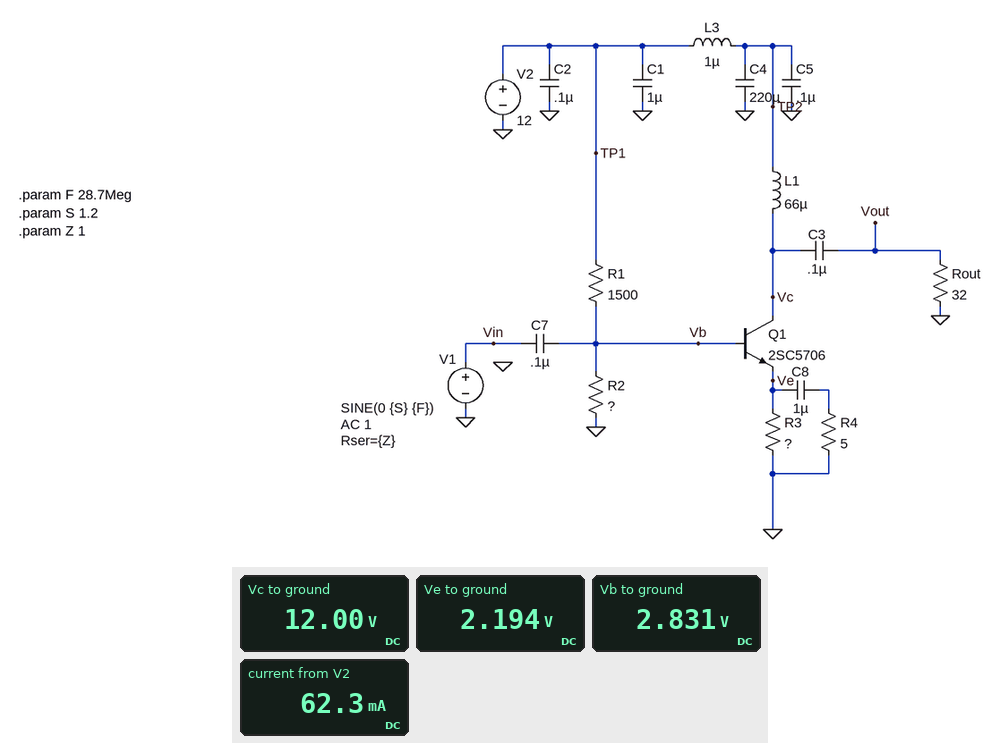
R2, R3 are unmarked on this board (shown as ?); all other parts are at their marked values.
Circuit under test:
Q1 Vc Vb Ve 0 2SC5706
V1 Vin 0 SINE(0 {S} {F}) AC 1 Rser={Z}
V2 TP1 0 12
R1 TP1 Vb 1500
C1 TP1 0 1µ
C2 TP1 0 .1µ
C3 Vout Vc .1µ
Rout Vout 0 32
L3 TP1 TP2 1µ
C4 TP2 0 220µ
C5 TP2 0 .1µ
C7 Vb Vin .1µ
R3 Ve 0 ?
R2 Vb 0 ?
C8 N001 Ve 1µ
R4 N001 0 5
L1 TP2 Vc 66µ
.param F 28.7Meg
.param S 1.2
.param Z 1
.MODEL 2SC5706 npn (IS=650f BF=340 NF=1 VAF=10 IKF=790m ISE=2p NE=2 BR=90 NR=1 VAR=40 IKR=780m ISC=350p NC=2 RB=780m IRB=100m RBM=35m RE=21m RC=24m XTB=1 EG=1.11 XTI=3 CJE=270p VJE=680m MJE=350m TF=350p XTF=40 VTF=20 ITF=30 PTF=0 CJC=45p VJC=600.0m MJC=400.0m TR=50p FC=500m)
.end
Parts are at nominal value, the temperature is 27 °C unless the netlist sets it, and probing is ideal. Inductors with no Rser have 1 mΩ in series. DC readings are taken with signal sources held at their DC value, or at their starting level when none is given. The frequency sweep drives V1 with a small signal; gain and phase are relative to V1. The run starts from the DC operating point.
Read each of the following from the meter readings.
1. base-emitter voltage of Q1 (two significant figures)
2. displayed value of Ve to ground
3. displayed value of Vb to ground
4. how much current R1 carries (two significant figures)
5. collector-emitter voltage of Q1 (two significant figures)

640 mV
2.194 V
2.831 V
6.1 mA
9.8 V
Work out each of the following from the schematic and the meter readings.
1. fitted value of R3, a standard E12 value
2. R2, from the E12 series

39 Ω
470 Ω
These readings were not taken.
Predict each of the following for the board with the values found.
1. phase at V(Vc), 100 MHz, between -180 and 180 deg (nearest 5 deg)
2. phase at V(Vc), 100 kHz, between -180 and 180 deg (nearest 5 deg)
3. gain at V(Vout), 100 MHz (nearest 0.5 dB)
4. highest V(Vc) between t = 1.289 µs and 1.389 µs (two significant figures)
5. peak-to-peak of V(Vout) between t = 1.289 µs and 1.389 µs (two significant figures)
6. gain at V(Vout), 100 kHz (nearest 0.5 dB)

130 deg
-140 deg
14.5 dB
14 V
9.3 V
16.0 dB
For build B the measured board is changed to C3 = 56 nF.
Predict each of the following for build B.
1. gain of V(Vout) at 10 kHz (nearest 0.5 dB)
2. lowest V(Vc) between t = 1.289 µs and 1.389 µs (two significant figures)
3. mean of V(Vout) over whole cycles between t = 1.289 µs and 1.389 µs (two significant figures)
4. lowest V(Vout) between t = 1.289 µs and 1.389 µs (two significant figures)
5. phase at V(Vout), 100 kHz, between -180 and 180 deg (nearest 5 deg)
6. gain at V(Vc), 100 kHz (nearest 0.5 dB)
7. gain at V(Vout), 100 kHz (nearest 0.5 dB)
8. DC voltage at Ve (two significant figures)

-29.5 dB
4.8 V
-470 mV
-6.5 V
-95 deg
20.0 dB
17.5 dB
2.2 V
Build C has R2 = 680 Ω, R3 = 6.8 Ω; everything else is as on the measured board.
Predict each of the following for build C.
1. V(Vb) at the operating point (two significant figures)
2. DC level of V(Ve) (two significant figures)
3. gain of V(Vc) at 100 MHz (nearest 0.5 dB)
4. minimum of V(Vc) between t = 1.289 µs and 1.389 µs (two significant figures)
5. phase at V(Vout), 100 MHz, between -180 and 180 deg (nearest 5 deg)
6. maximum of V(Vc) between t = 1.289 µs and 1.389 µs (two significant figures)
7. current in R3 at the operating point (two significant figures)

3.4 V
2.7 V
18.5 dB
3.2 V
135 deg
24 V
390 mA
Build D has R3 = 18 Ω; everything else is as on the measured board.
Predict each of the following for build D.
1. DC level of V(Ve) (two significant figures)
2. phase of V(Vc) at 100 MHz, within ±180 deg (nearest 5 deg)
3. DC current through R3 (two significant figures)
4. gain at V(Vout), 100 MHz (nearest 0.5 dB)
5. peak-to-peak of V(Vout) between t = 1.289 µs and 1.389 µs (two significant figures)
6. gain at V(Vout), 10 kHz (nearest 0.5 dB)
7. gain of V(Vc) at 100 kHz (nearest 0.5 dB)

2.1 V
135 deg
120 mA
16.0 dB
12 V
-22.5 dB
18.0 dB
